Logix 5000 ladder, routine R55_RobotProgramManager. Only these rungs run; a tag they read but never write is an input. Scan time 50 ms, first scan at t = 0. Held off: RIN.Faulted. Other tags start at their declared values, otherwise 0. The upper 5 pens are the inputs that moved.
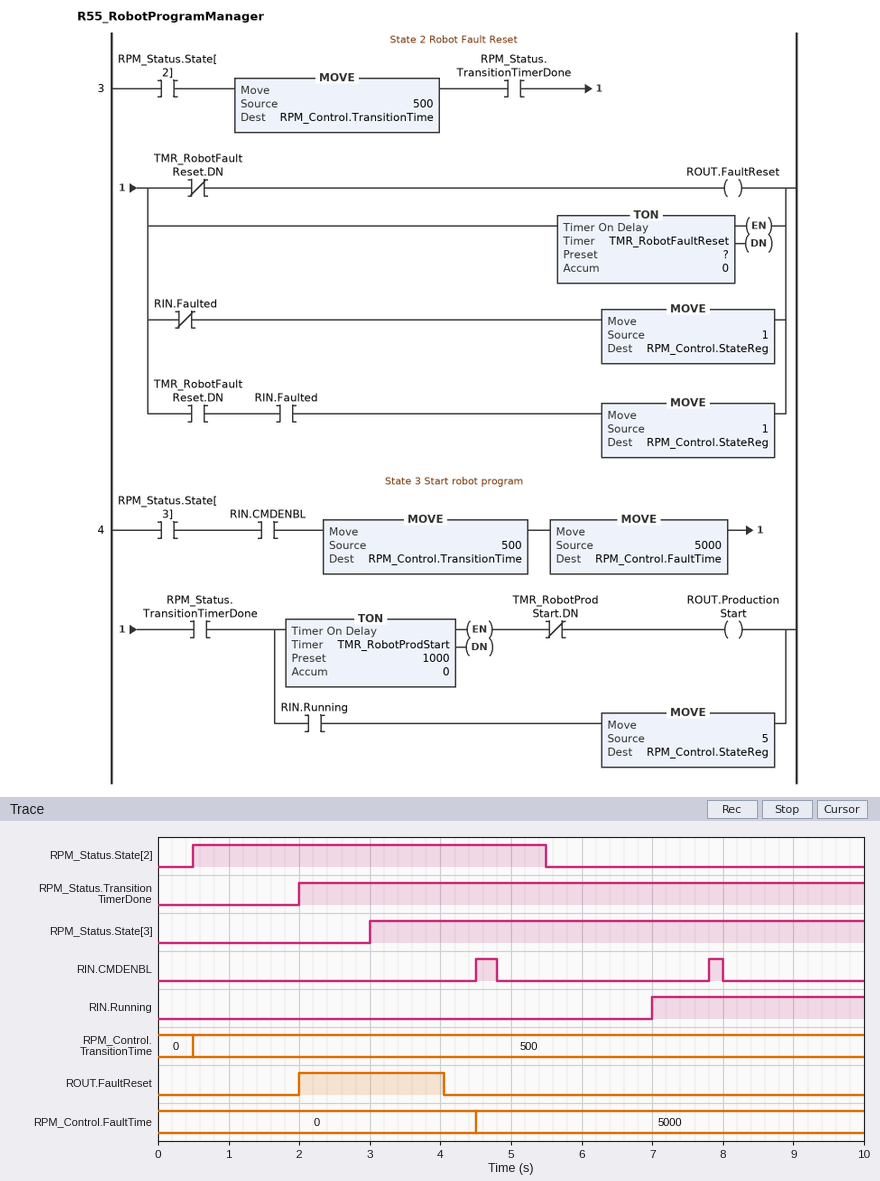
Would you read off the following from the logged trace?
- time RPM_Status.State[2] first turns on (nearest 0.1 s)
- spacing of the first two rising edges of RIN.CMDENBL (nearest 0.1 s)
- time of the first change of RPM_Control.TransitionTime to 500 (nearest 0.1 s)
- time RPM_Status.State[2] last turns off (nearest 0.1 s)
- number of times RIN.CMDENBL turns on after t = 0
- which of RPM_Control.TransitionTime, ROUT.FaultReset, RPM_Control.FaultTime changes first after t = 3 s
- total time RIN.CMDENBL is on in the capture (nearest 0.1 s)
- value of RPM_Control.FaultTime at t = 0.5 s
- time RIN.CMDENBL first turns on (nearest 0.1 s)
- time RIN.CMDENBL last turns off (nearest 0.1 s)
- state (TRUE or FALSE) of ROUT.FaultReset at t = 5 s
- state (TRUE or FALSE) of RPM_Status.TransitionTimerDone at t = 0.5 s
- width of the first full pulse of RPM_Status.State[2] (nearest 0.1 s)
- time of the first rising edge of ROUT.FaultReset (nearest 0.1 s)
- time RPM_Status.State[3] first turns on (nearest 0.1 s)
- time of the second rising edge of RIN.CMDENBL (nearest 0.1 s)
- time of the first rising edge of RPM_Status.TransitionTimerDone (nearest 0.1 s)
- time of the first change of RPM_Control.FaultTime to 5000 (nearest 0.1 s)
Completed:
0.5 s
3.3 s
0.5 s
5.5 s
2
ROUT.FaultReset
0.5 s
0
4.5 s
8.0 s
FALSE
FALSE
5.0 s
2.0 s
3.0 s
7.8 s
2.0 s
4.5 s
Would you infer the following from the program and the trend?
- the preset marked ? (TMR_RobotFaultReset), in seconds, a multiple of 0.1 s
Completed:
2.0 s
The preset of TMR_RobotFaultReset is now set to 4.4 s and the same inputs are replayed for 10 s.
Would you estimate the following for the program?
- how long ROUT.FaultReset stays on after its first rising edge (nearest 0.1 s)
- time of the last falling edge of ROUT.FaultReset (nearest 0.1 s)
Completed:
3.5 s
5.5 s
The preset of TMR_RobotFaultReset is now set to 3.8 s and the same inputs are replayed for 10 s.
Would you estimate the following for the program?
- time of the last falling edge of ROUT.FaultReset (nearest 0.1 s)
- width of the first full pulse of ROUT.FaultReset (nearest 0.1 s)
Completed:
5.5 s
3.5 s
